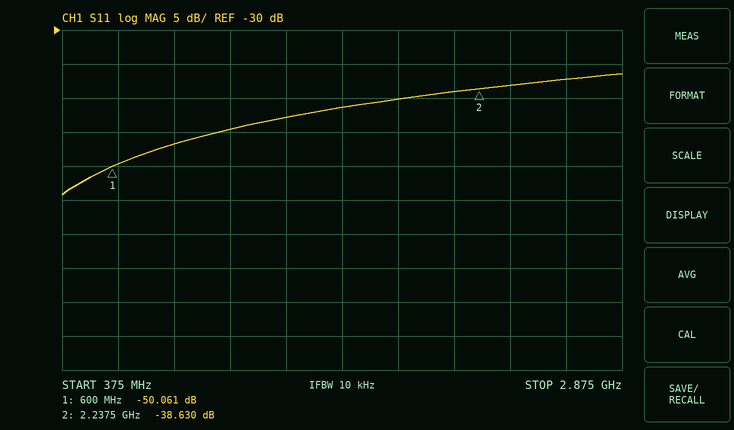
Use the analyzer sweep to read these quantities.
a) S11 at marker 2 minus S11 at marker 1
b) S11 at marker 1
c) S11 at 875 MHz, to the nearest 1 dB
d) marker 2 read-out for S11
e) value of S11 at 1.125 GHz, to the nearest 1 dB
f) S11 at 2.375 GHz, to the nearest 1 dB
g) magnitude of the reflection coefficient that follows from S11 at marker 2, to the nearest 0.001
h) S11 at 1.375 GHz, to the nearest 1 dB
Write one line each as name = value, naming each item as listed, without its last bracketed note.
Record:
S11 at marker 2 minus S11 at marker 1 = 11.431 dB
S11 at marker 1 = -50.061 dB
S11 at 875 MHz, to the nearest 1 dB = -47 dB
marker 2 read-out for S11 = -38.630 dB
value of S11 at 1.125 GHz, to the nearest 1 dB = -45 dB
S11 at 2.375 GHz, to the nearest 1 dB = -38 dB
magnitude of the reflection coefficient that follows from S11 at marker 2, to the nearest 0.001 = 0.012
S11 at 1.375 GHz, to the nearest 1 dB = -43 dB
